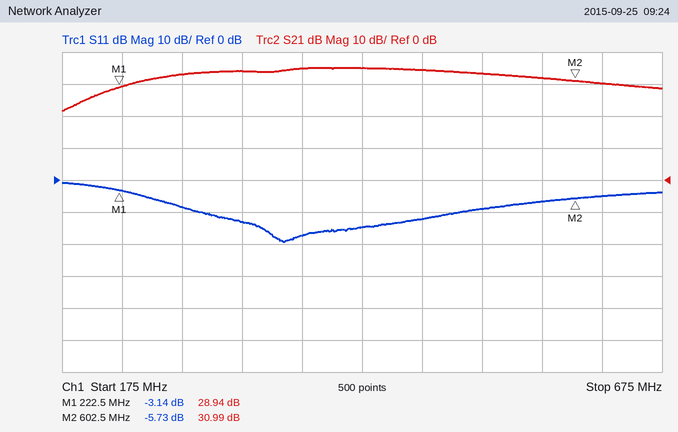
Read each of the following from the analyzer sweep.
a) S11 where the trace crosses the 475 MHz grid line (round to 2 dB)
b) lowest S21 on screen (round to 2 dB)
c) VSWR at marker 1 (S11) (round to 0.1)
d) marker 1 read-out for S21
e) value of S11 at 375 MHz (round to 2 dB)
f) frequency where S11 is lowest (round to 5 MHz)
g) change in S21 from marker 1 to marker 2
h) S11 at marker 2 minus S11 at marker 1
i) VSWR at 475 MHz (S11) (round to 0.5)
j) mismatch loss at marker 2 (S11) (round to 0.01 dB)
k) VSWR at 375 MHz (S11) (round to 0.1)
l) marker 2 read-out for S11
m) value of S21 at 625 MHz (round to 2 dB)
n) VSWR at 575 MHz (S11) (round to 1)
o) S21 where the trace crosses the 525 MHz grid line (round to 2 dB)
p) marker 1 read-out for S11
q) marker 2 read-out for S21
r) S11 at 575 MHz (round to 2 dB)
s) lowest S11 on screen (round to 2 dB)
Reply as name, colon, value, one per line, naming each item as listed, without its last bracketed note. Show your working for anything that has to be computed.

S11 where the trace crosses the 475 MHz grid line: -12 dB
lowest S21 on screen: 22 dB
VSWR at marker 1 (S11): (1 + 0.6966)/(1 − 0.6966) ≈ 5.6
marker 1 read-out for S21: 28.94 dB
value of S11 at 375 MHz: -18 dB
frequency where S11 is lowest: 360 MHz
change in S21 from marker 1 to marker 2: 30.99 − (28.94) = 2.05 dB
S11 at marker 2 minus S11 at marker 1: -5.73 − (-3.14) = -2.59 dB
VSWR at 475 MHz (S11): |Γ| = 10^(-12/20) = 0.2512; VSWR = (1 + 0.2512)/(1 − 0.2512) ≈ 1.67, so 1.5 to the nearest 0.5
mismatch loss at marker 2 (S11): −10 log10(1 − 10^(-5.73/10)) ≈ 1.35 dB
VSWR at 375 MHz (S11): |Γ| = 10^(-18/20) = 0.1259; VSWR = (1 + 0.1259)/(1 − 0.1259) ≈ 1.3
marker 2 read-out for S11: -5.73 dB
value of S21 at 625 MHz: 30 dB
VSWR at 575 MHz (S11): |Γ| = 10^(-6/20) = 0.5012; VSWR = (1 + 0.5012)/(1 − 0.5012) ≈ 3
S21 where the trace crosses the 525 MHz grid line: 34 dB
marker 1 read-out for S11: -3.14 dB
marker 2 read-out for S21: 30.99 dB
S11 at 575 MHz: -6 dB
lowest S11 on screen: -20 dB
